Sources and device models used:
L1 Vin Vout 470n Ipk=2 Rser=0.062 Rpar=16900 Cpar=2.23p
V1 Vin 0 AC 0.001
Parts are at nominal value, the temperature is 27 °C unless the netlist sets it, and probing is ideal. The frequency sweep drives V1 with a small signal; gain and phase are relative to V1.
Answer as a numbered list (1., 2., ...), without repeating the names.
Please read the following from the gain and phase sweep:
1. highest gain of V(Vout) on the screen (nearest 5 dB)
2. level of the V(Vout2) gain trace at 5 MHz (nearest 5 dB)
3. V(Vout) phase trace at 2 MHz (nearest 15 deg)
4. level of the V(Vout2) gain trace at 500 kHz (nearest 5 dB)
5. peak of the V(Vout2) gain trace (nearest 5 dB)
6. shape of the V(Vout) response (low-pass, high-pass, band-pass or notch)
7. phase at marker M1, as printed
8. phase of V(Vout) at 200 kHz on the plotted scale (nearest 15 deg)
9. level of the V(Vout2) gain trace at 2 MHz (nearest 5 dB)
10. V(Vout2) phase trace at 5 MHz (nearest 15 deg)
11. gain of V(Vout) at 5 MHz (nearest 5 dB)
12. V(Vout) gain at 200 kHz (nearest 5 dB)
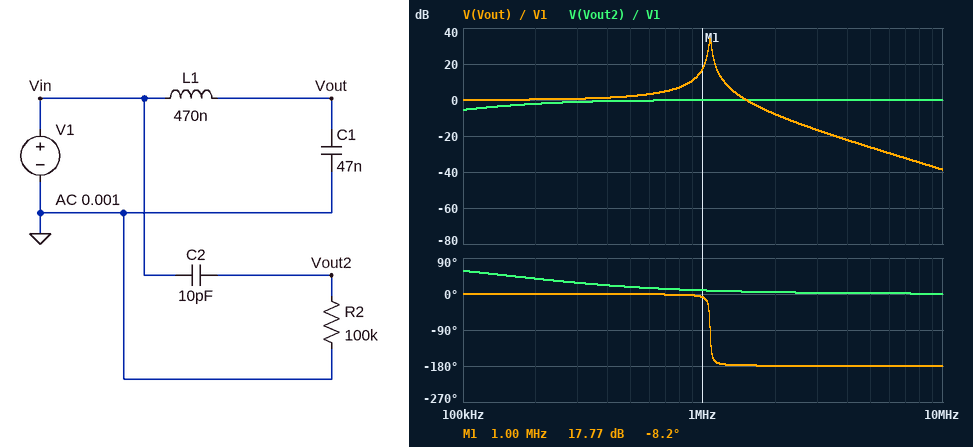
1. 35 dB
2. 0 dB
3. -180 deg
4. 0 dB
5. 0 dB
6. low-pass
7. -8.2 deg
8. 0 deg
9. 0 dB
10. 0 deg
11. -25 dB
12. 0 dB
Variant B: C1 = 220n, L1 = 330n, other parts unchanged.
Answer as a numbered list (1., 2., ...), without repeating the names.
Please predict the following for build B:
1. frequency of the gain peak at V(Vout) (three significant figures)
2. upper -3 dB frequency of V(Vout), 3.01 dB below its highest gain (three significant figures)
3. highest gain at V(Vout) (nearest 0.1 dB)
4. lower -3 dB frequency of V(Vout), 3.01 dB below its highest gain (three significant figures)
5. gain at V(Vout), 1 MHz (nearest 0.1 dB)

1. 590 kHz
2. 605 kHz
3. 25.9 dB
4. 575 kHz
5. -5.4 dB
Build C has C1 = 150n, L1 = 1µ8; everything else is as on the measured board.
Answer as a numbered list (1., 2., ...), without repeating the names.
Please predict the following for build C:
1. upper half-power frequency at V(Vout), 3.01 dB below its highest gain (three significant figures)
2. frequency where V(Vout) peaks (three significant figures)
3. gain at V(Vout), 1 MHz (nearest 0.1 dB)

1. 309 kHz
2. 306 kHz
3. -19.7 dB
